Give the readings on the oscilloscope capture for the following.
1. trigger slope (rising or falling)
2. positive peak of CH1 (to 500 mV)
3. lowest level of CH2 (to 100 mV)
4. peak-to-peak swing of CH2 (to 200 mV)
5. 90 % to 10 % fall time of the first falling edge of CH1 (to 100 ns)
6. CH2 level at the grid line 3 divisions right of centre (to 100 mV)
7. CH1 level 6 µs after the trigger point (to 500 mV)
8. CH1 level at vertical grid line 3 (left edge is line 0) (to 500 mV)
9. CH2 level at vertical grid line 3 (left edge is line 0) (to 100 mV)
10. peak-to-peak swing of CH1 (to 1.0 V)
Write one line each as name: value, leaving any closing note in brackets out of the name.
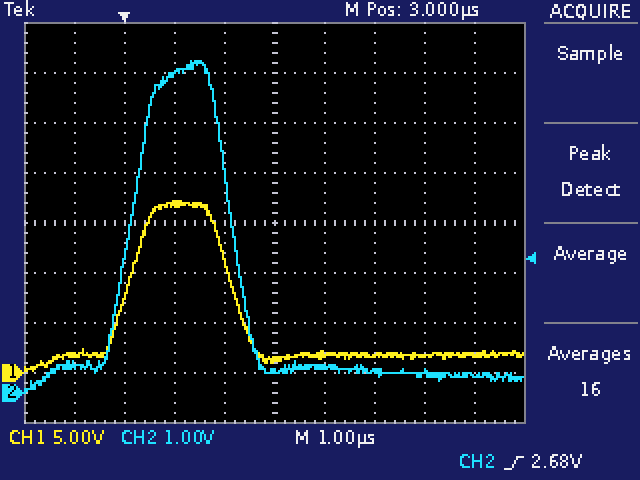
trigger slope: rising
positive peak of CH1: 17.0 V
lowest level of CH2: 0.0 V
peak-to-peak swing of CH2: 6.6 V
90 % to 10 % fall time of the first falling edge of CH1: 800 ns
CH2 level at the grid line 3 divisions right of centre: 400 mV
CH1 level 6 µs after the trigger point: 1.5 V
CH1 level at vertical grid line 3 (left edge is line 0): 17.0 V
CH2 level at vertical grid line 3 (left edge is line 0): 6.4 V
peak-to-peak swing of CH1: 17.0 V
